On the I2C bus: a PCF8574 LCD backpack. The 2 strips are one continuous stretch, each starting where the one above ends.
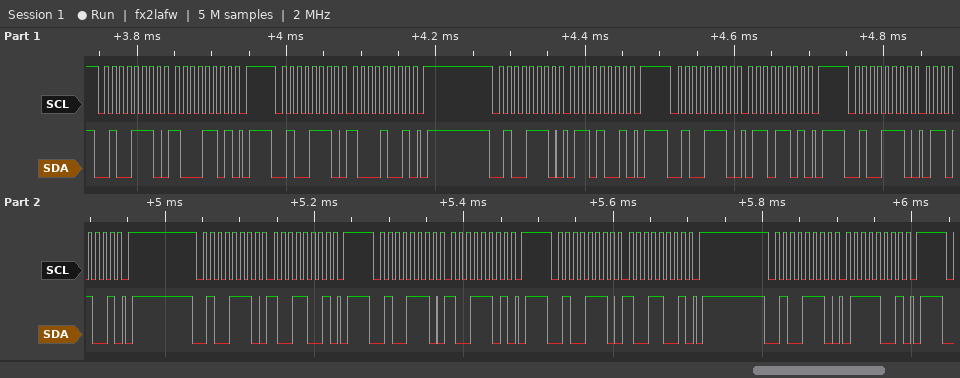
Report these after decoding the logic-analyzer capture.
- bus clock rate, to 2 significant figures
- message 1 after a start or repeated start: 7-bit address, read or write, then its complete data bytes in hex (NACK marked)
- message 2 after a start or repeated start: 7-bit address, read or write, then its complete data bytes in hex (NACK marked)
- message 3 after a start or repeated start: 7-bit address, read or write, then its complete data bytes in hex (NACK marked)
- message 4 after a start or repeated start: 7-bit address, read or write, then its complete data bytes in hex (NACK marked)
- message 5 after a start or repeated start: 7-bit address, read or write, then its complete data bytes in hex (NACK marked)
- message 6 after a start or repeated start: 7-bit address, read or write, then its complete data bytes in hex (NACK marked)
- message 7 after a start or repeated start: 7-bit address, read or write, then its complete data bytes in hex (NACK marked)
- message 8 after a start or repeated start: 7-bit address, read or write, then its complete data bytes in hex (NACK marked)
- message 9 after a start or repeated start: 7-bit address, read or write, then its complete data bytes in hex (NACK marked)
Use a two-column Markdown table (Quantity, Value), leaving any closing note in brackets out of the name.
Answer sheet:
| Quantity | Value |
|---|---|
| bus clock rate, to 2 significant figures | 100 kHz |
| message 1 after a start or repeated start: 7-bit address, read or write, then its complete data bytes in hex | 0x27 write: 8D |
| message 2 after a start or repeated start: 7-bit address, read or write, then its complete data bytes in hex | 0x27 write: 89 |
| message 3 after a start or repeated start: 7-bit address, read or write, then its complete data bytes in hex | 0x27 write: 69 |
| message 4 after a start or repeated start: 7-bit address, read or write, then its complete data bytes in hex | 0x27 write: 6D |
| message 5 after a start or repeated start: 7-bit address, read or write, then its complete data bytes in hex | 0x27 write: 69 |
| message 6 after a start or repeated start: 7-bit address, read or write, then its complete data bytes in hex | 0x27 write: 99 |
| message 7 after a start or repeated start: 7-bit address, read or write, then its complete data bytes in hex | 0x27 write: 9D |
| message 8 after a start or repeated start: 7-bit address, read or write, then its complete data bytes in hex | 0x27 write: 99 |
| message 9 after a start or repeated start: 7-bit address, read or write, then its complete data bytes in hex | 0x27 write: 79 |
